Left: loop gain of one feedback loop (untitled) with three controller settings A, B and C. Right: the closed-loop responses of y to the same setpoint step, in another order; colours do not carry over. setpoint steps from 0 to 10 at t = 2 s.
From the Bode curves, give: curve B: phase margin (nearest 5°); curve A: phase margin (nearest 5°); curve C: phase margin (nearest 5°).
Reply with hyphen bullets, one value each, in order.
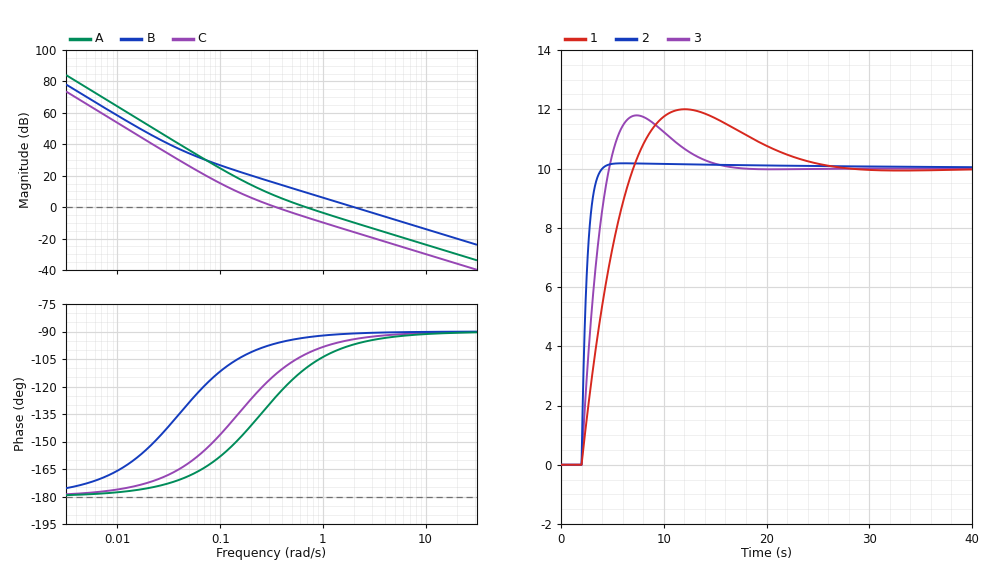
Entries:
- 90°
- 70°
- 65°
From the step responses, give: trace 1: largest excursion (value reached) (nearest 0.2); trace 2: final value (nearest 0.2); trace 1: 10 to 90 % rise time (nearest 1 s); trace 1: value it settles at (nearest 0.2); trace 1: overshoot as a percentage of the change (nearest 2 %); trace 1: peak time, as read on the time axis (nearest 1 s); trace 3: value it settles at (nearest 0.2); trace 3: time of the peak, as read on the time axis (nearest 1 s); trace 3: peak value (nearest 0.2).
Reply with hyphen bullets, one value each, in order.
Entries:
- 12.0
- 10.0
- 4 s
- 10.0
- 20 %
- 12 s
- 10.0
- 7 s
- 11.8
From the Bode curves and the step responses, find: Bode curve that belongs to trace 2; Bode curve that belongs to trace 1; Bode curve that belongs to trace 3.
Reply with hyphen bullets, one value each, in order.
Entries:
- B
- C
- A
